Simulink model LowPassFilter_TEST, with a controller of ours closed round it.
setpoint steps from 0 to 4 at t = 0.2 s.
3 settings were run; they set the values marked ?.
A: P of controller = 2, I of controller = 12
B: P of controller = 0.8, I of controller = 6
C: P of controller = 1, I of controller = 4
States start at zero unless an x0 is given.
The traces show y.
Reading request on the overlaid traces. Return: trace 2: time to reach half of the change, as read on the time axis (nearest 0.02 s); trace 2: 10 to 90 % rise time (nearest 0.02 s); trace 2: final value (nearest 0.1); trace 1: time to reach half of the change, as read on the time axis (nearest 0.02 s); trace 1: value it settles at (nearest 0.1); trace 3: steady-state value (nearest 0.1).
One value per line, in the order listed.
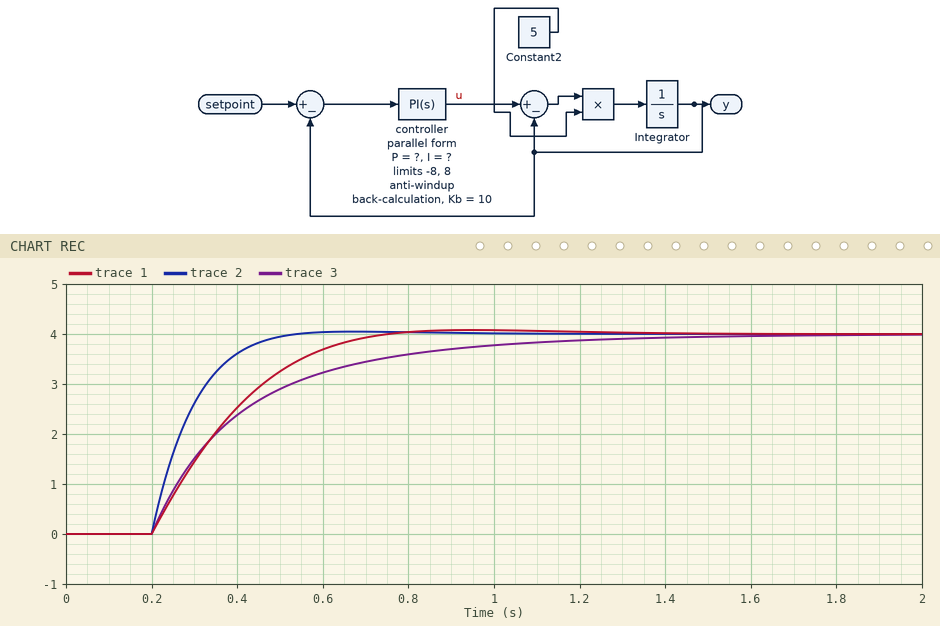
0.26 s
0.18 s
4.0
0.34 s
4.0
4.0
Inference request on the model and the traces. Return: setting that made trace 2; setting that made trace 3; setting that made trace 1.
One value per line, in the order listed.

A
C
B
